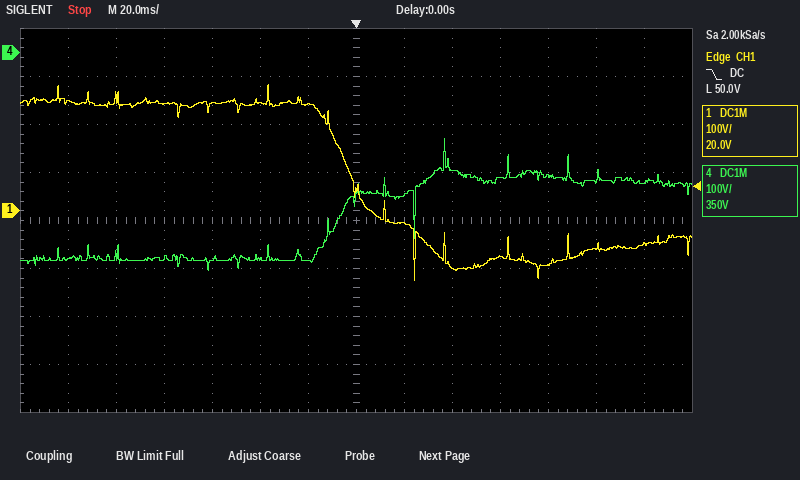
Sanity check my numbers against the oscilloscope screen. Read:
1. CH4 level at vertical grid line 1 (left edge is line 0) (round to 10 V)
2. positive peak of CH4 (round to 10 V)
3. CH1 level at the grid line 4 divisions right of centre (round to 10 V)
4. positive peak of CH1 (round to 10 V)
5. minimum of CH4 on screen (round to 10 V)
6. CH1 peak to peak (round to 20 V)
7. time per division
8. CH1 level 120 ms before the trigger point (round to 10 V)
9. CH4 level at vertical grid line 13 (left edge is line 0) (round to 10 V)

-430 V
-180 V
-110 V
260 V
-450 V
400 V
20 ms
230 V
-270 V
